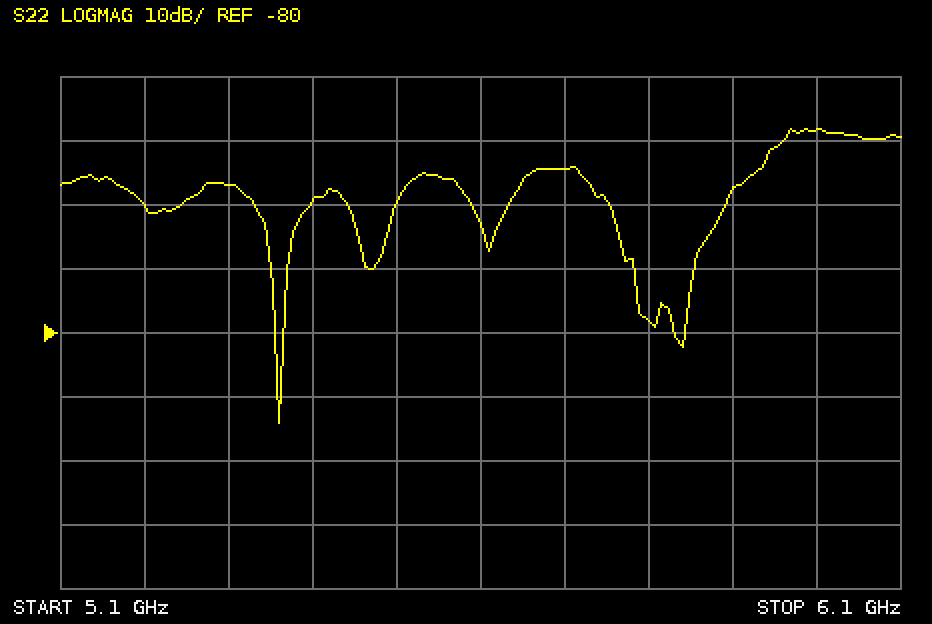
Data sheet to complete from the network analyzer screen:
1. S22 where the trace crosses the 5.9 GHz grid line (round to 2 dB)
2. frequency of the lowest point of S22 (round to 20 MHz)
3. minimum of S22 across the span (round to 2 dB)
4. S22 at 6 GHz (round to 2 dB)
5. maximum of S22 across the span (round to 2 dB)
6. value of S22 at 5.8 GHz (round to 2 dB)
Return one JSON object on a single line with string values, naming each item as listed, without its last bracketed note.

{"S22 where the trace crosses the 5.9 GHz grid line": "-58 dB", "frequency of the lowest point of S22": "5.36 GHz", "minimum of S22 across the span": "-94 dB", "S22 at 6 GHz": "-48 dB", "maximum of S22 across the span": "-48 dB", "value of S22 at 5.8 GHz": "-78 dB"}
